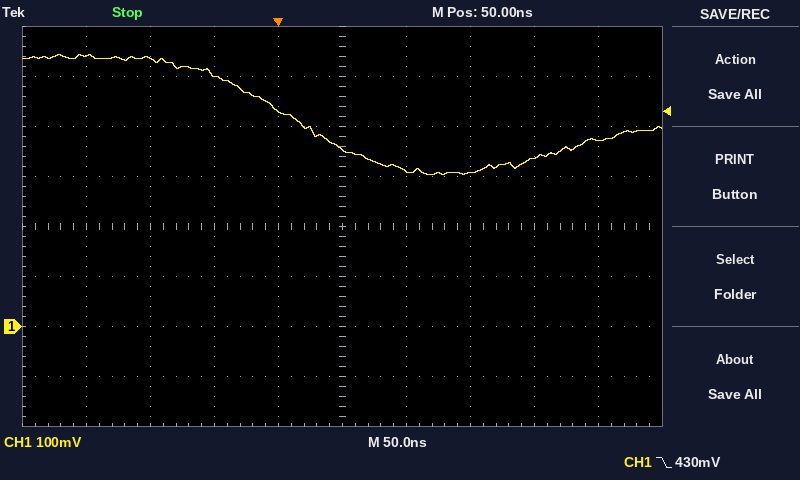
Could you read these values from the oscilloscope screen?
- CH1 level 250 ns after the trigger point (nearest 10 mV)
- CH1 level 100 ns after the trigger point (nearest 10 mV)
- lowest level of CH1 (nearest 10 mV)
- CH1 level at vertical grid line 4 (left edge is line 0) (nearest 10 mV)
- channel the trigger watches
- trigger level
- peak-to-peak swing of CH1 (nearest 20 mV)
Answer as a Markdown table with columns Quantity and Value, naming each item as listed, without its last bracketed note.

| Quantity | Value |
|---|---|
| CH1 level 250 ns after the trigger point | 370 mV |
| CH1 level 100 ns after the trigger point | 310 mV |
| lowest level of CH1 | 300 mV |
| CH1 level at vertical grid line 4 (left edge is line 0) | 430 mV |
| channel the trigger watches | CH1 |
| trigger level | 430 mV |
| peak-to-peak swing of CH1 | 240 mV |
